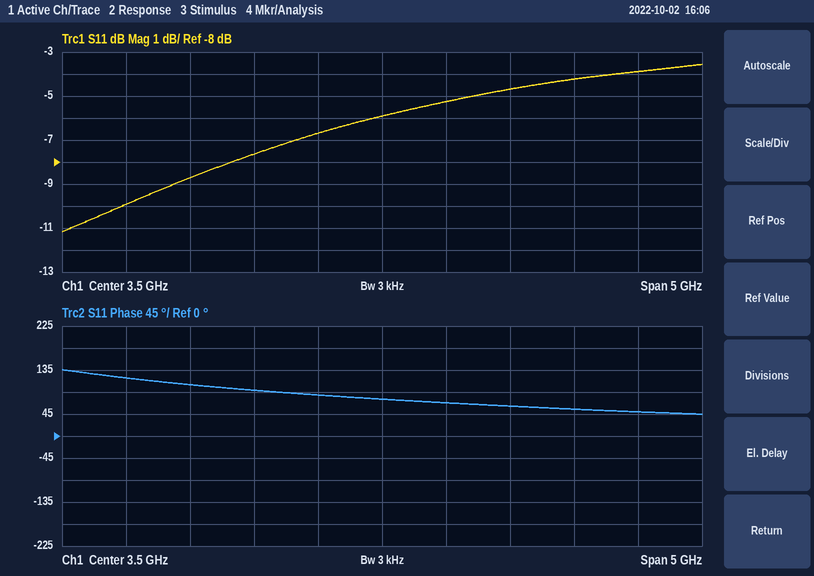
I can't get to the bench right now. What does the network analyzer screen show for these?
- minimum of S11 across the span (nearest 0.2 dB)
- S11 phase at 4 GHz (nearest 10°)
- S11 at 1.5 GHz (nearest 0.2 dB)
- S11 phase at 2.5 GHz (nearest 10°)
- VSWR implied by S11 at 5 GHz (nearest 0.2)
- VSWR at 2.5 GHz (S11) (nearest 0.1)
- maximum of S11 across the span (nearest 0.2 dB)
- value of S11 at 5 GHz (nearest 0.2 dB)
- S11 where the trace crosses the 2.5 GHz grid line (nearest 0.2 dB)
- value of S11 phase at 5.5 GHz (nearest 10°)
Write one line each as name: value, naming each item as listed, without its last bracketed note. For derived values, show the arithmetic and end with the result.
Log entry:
minimum of S11 across the span: -11.2 dB
S11 phase at 4 GHz: 70°
S11 at 1.5 GHz: -10.0 dB
S11 phase at 2.5 GHz: 90°
VSWR implied by S11 at 5 GHz: |Γ| = 10^(-4.2/20) = 0.6166; VSWR = (1 + 0.6166)/(1 − 0.6166) ≈ 4.2
VSWR at 2.5 GHz (S11): |Γ| = 10^(-7.6/20) = 0.4169; VSWR = (1 + 0.4169)/(1 − 0.4169) ≈ 2.4
maximum of S11 across the span: -3.6 dB
value of S11 at 5 GHz: -4.2 dB
S11 where the trace crosses the 2.5 GHz grid line: -7.6 dB
value of S11 phase at 5.5 GHz: 50°
